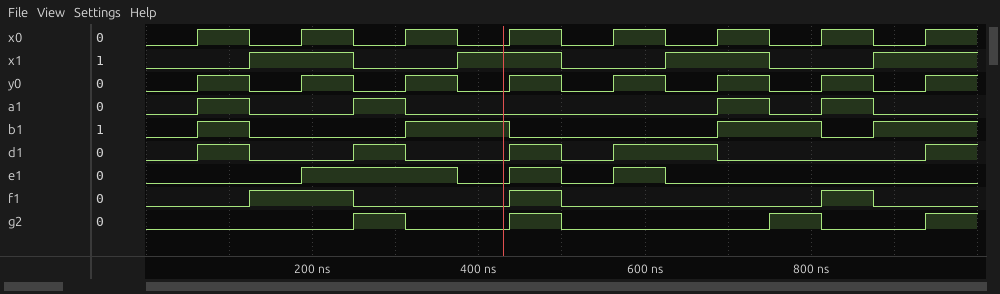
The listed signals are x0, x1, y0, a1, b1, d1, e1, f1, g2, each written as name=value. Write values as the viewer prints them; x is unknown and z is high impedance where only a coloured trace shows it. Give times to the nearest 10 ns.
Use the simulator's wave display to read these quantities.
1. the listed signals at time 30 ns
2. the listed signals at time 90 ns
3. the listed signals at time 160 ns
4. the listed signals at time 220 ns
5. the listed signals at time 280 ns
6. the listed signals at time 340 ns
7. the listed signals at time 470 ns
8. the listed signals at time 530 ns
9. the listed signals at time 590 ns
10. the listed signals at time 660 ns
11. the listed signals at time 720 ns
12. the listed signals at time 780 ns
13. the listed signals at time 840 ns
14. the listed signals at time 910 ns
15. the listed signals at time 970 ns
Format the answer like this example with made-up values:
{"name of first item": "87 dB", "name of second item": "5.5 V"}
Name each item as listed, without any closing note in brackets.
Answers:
{"the listed signals at time 30 ns": "x0=0, x1=0, y0=0, a1=0, b1=0, d1=0, e1=0, f1=0, g2=0", "the listed signals at time 90 ns": "x0=1, x1=0, y0=1, a1=1, b1=1, d1=1, e1=0, f1=0, g2=0", "the listed signals at time 160 ns": "x0=0, x1=1, y0=0, a1=0, b1=0, d1=0, e1=0, f1=1, g2=0", "the listed signals at time 220 ns": "x0=1, x1=1, y0=1, a1=0, b1=0, d1=0, e1=1, f1=1, g2=0", "the listed signals at time 280 ns": "x0=0, x1=0, y0=0, a1=1, b1=0, d1=1, e1=1, f1=0, g2=1", "the listed signals at time 340 ns": "x0=1, x1=0, y0=1, a1=0, b1=1, d1=0, e1=1, f1=0, g2=0", "the listed signals at time 470 ns": "x0=1, x1=1, y0=1, a1=0, b1=0, d1=1, e1=1, f1=1, g2=1", "the listed signals at time 530 ns": "x0=0, x1=0, y0=0, a1=0, b1=0, d1=0, e1=0, f1=0, g2=0", "the listed signals at time 590 ns": "x0=1, x1=0, y0=1, a1=0, b1=0, d1=1, e1=1, f1=0, g2=0", "the listed signals at time 660 ns": "x0=0, x1=1, y0=0, a1=0, b1=0, d1=1, e1=0, f1=0, g2=0", "the listed signals at time 720 ns": "x0=1, x1=1, y0=1, a1=1, b1=1, d1=0, e1=0, f1=0, g2=0", "the listed signals at time 780 ns": "x0=0, x1=0, y0=0, a1=0, b1=1, d1=0, e1=0, f1=0, g2=1", "the listed signals at time 840 ns": "x0=1, x1=0, y0=1, a1=1, b1=0, d1=0, e1=0, f1=1, g2=0", "the listed signals at time 910 ns": "x0=0, x1=1, y0=0, a1=0, b1=1, d1=0, e1=0, f1=0, g2=0", "the listed signals at time 970 ns": "x0=1, x1=1, y0=1, a1=0, b1=1, d1=1, e1=0, f1=0, g2=1"}
